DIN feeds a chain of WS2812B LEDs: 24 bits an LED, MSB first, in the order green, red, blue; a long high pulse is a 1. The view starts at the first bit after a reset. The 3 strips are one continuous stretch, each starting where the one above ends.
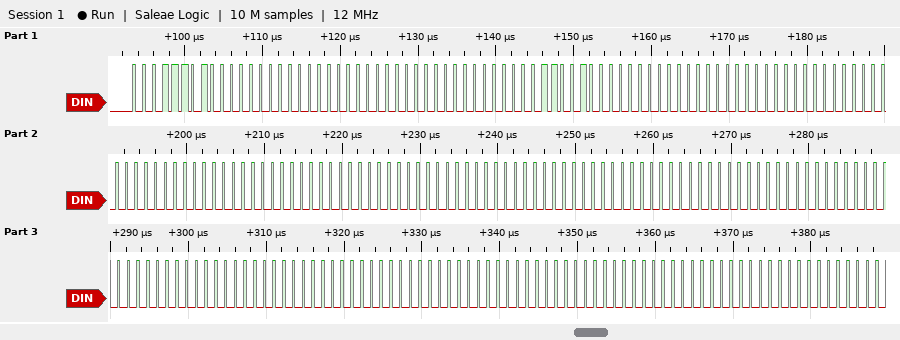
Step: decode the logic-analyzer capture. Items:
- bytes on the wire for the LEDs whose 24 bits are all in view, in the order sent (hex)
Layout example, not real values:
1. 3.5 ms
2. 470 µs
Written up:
1. 1D 00 00 00 00 32 00 00 00 00 00 00 00 00 00 00 00 00 00 00 00 00 00 00 00 00 00
